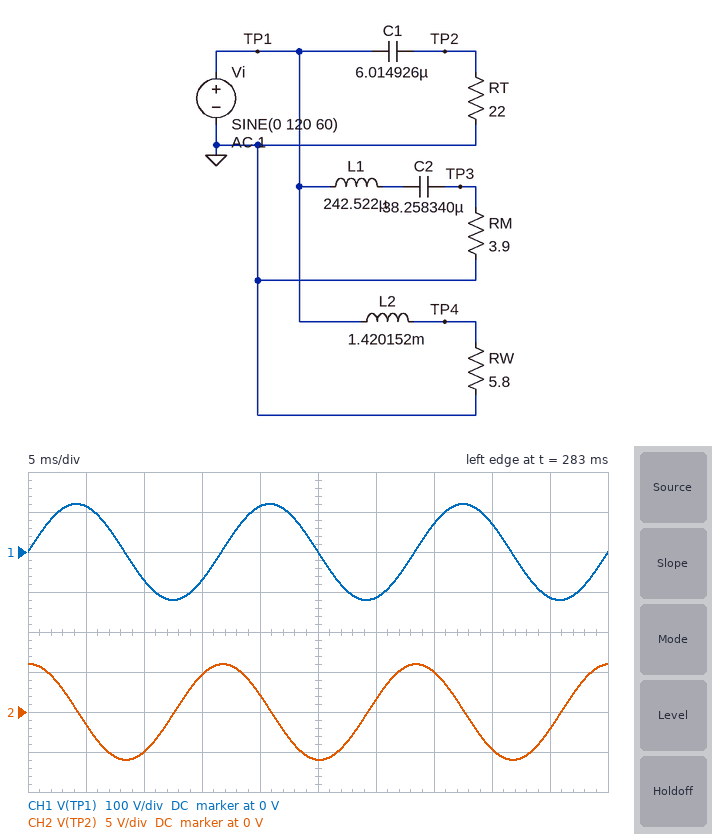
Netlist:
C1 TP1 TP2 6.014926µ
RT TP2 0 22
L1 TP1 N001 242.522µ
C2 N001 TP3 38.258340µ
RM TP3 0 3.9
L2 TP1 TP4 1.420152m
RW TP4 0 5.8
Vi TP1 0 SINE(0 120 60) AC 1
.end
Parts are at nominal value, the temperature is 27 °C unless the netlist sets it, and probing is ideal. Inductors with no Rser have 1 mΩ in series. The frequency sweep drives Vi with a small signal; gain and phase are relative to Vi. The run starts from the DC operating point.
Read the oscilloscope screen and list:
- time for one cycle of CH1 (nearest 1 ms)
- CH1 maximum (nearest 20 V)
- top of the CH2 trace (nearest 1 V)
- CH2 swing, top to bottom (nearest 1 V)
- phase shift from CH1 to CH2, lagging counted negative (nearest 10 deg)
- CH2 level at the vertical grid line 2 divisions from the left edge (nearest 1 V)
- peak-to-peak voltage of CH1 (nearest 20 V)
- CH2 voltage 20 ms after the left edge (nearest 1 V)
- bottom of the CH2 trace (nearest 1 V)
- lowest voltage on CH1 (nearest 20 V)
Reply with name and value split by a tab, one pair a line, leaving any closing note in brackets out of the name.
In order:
time for one cycle of CH1	17 ms
CH1 maximum	120 V
top of the CH2 trace	6 V
CH2 swing, top to bottom	12 V
phase shift from CH1 to CH2, lagging counted negative	90 deg
CH2 level at the vertical grid line 2 divisions from the left edge	-5 V
peak-to-peak voltage of CH1	240 V
CH2 voltage 20 ms after the left edge	2 V
bottom of the CH2 trace	-6 V
lowest voltage on CH1	-120 V
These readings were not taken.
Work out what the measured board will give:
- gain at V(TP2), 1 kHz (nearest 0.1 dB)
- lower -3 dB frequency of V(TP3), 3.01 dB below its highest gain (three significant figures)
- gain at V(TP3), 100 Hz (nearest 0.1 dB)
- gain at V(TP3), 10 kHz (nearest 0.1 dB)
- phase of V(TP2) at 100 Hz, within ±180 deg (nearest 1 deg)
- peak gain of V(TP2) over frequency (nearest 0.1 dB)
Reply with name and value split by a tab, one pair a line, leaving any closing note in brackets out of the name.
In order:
gain at V(TP2), 1 kHz	-3.9 dB
lower -3 dB frequency of V(TP3), 3.01 dB below its highest gain	810 Hz
gain at V(TP3), 100 Hz	-20.6 dB
gain at V(TP3), 10 kHz	-11.9 dB
phase of V(TP2) at 100 Hz, within ±180 deg	85 deg
peak gain of V(TP2) over frequency	0 dB
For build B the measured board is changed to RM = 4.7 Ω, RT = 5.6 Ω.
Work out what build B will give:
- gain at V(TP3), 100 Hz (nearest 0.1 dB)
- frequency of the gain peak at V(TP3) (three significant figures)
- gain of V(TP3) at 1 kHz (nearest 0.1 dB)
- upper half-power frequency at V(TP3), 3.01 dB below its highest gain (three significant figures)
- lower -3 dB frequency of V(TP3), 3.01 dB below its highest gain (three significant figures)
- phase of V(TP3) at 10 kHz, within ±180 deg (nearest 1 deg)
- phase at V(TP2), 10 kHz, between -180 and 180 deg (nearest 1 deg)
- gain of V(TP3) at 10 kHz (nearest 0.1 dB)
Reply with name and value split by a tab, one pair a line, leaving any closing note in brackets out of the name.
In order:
gain at V(TP3), 100 Hz	-19.0 dB
frequency of the gain peak at V(TP3)	1.65 kHz
gain of V(TP3) at 1 kHz	-1.2 dB
upper half-power frequency at V(TP3), 3.01 dB below its highest gain	3.80 kHz
lower -3 dB frequency of V(TP3), 3.01 dB below its highest gain	718 Hz
phase of V(TP3) at 10 kHz, within ±180 deg	-72 deg
phase at V(TP2), 10 kHz, between -180 and 180 deg	25 deg
gain of V(TP3) at 10 kHz	-10.4 dB
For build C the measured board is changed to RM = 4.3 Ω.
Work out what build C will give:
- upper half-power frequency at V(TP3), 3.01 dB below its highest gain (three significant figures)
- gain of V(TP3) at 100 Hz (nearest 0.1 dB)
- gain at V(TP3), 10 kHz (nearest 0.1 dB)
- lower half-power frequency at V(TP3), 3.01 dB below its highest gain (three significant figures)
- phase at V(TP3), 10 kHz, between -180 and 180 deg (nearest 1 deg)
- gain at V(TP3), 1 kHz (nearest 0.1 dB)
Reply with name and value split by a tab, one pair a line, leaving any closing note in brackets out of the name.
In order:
upper half-power frequency at V(TP3), 3.01 dB below its highest gain	3.58 kHz
gain of V(TP3) at 100 Hz	-19.7 dB
gain at V(TP3), 10 kHz	-11.1 dB
lower half-power frequency at V(TP3), 3.01 dB below its highest gain	762 Hz
phase at V(TP3), 10 kHz, between -180 and 180 deg	-74 deg
gain at V(TP3), 1 kHz	-1.4 dB
